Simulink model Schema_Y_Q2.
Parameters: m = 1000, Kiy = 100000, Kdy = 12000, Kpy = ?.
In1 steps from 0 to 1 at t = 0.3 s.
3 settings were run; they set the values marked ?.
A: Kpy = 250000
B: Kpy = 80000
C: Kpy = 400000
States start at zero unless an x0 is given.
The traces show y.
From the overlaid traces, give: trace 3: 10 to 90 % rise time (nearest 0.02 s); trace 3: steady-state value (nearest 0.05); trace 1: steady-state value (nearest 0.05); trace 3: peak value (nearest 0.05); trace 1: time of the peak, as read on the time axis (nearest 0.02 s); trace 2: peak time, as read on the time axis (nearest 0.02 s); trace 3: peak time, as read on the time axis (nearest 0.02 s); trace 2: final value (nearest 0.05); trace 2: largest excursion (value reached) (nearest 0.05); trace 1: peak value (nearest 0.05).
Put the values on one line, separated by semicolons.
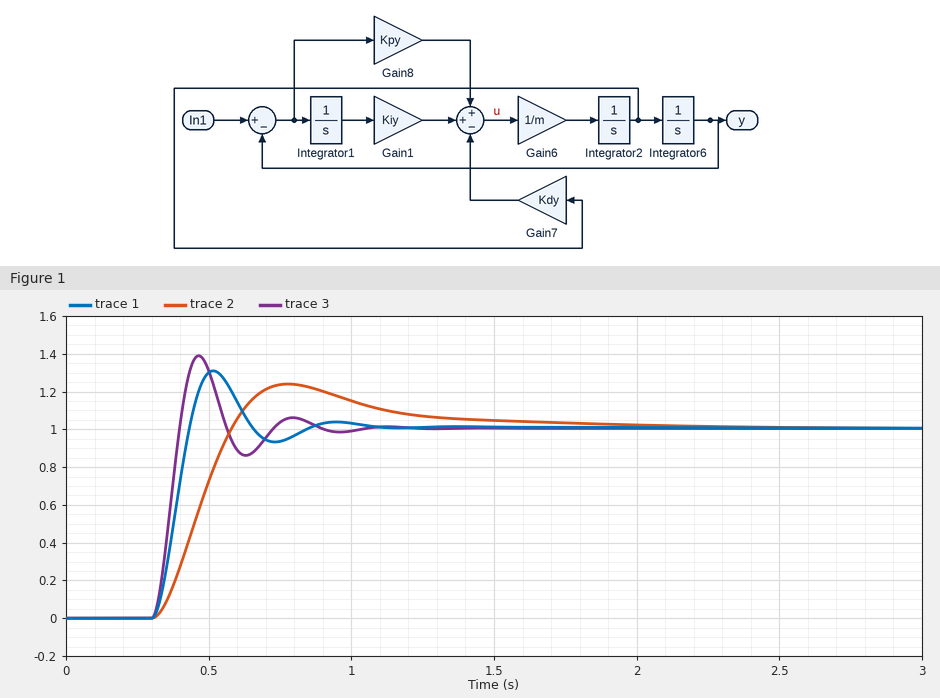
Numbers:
0.06 s; 1.00; 1.00; 1.40; 0.52 s; 0.78 s; 0.46 s; 1.00; 1.25; 1.30
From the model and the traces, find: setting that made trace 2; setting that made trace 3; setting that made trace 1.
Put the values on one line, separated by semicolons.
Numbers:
B; C; A
